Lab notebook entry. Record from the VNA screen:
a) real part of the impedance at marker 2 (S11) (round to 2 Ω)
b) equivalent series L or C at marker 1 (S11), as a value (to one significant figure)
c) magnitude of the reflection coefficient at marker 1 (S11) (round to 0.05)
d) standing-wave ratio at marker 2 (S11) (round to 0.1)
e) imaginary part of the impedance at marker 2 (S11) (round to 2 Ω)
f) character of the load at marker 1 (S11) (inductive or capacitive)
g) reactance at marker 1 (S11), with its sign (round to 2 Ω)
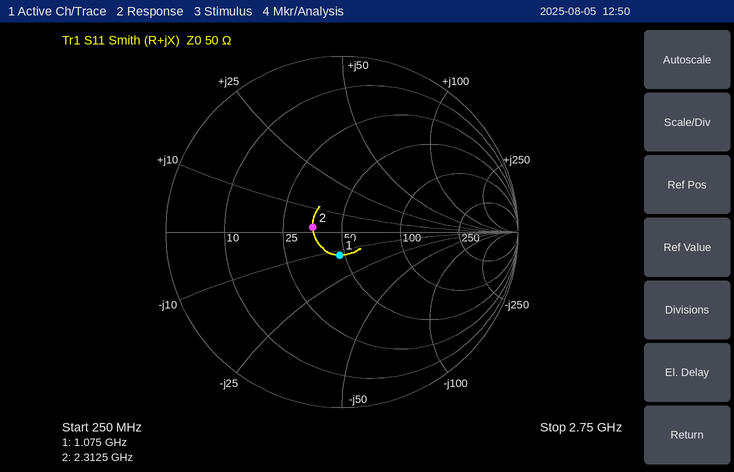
36 Ω
10 pF
0.15
1.4
+2 Ω
capacitive
-12 Ω
